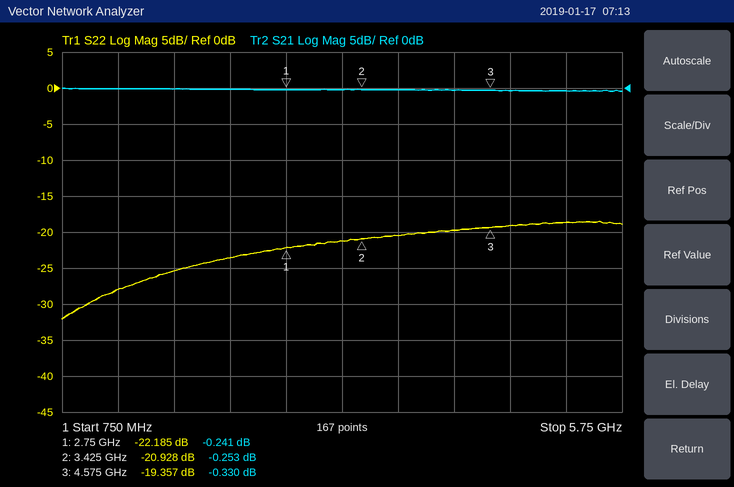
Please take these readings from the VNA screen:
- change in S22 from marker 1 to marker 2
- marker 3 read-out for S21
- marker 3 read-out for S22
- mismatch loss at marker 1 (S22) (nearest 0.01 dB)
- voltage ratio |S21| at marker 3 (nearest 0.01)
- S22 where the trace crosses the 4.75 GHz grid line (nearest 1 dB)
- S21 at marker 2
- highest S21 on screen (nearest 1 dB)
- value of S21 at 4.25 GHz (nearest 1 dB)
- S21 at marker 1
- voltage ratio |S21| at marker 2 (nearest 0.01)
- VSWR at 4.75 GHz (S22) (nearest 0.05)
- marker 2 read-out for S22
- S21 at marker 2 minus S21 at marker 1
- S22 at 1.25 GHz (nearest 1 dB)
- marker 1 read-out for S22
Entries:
1.257 dB
-0.330 dB
-19.357 dB
0.03 dB
0.96
-19 dB
-0.253 dB
0 dB
0 dB
-0.241 dB
0.97
1.25
-20.928 dB
-0.012 dB
-28 dB
-22.185 dB
